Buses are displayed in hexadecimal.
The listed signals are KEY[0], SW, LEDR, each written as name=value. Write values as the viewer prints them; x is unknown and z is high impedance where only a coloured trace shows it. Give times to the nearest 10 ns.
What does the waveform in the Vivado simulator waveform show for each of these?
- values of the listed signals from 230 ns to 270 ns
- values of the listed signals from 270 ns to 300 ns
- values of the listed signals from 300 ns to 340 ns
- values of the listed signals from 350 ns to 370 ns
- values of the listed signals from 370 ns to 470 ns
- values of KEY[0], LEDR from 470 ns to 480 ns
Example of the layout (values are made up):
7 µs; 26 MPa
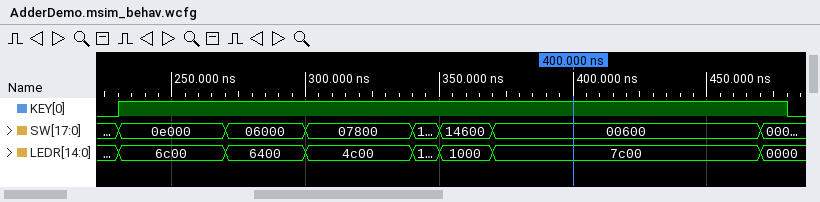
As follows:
KEY[0]=1, SW=0e000, LEDR=6c00; KEY[0]=1, SW=06000, LEDR=6400; KEY[0]=1, SW=07800, LEDR=4c00; KEY[0]=1, SW=14600, LEDR=1000; KEY[0]=1, SW=00600, LEDR=7c00; KEY[0]=1, LEDR=0000
